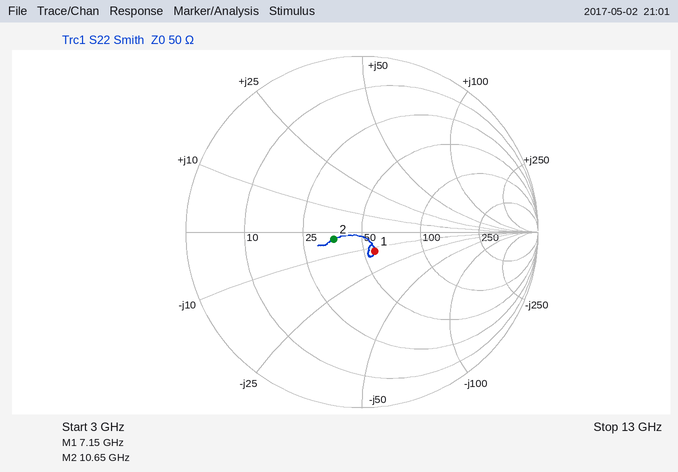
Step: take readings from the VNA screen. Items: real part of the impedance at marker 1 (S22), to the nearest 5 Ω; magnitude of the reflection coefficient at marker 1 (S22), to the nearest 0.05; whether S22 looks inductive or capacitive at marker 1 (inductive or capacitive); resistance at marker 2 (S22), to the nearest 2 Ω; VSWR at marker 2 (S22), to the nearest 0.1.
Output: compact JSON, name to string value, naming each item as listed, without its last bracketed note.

{"real part of the impedance at marker 1 (S22), to the nearest 5 Ω": "55 Ω", "magnitude of the reflection coefficient at marker 1 (S22), to the nearest 0.05": "0.15", "whether S22 looks inductive or capacitive at marker 1": "capacitive", "resistance at marker 2 (S22), to the nearest 2 Ω": "36 Ω", "VSWR at marker 2 (S22), to the nearest 0.1": "1.4"}
